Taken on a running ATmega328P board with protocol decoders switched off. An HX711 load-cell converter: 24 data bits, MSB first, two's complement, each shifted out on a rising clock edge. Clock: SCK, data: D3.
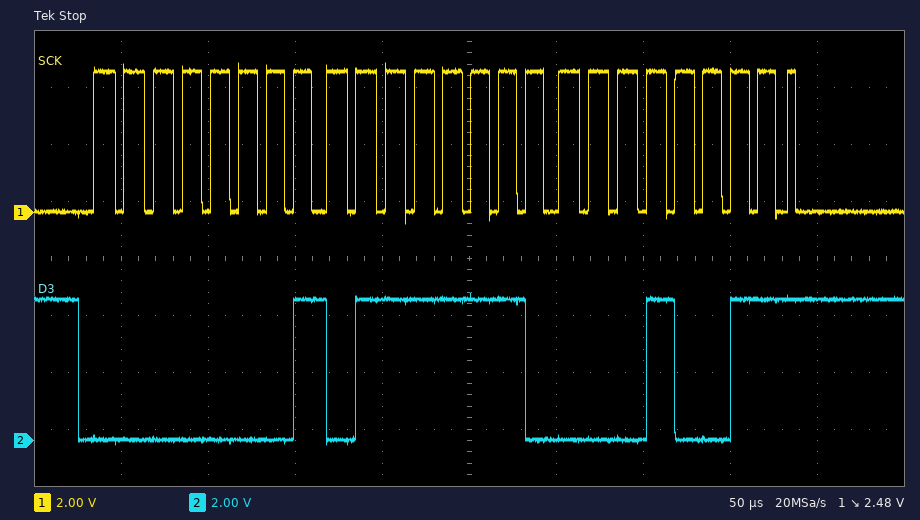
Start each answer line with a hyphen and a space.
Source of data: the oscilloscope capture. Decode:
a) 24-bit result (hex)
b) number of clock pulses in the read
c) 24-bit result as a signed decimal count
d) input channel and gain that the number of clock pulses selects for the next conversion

- 0x017E13
- 25
- 97811
- channel A, gain 128
